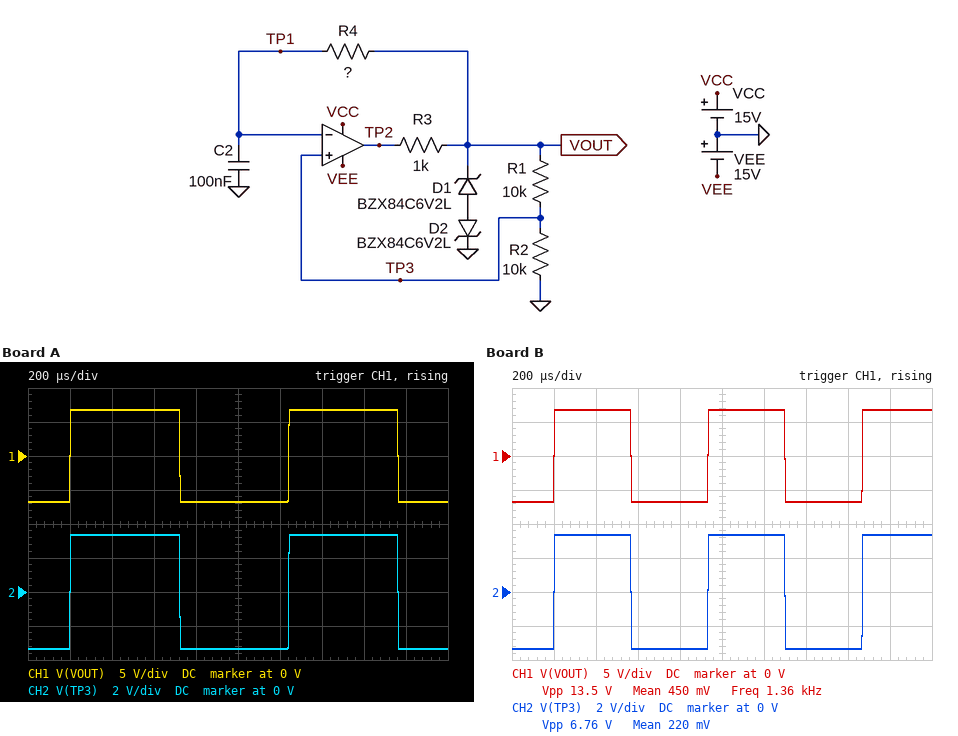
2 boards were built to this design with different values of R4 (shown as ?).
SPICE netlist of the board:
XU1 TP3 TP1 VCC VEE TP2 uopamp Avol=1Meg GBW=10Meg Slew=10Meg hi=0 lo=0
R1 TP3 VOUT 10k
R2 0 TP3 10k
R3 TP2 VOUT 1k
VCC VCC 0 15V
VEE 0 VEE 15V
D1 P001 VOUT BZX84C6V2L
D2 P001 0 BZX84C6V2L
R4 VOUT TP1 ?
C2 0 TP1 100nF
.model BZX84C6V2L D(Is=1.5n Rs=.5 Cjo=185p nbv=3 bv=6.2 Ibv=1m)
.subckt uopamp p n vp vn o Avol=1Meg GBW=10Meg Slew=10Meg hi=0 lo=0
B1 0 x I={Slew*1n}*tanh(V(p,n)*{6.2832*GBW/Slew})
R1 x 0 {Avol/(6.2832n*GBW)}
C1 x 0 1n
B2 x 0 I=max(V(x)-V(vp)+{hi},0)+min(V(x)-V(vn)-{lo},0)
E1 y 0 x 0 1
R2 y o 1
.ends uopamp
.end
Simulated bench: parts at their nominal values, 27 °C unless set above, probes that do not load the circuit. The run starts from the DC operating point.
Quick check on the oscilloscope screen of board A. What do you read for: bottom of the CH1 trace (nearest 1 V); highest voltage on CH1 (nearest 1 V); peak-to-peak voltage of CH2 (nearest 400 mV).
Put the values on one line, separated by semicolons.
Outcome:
-7 V; 7 V; 6.8 V
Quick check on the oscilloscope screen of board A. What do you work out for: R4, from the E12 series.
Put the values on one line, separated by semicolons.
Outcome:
4.7 kΩ
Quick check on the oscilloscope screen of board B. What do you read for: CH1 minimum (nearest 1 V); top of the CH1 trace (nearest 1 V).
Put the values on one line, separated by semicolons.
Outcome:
-7 V; 7 V
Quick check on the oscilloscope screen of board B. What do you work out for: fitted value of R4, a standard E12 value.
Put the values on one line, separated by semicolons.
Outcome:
3.3 kΩ
